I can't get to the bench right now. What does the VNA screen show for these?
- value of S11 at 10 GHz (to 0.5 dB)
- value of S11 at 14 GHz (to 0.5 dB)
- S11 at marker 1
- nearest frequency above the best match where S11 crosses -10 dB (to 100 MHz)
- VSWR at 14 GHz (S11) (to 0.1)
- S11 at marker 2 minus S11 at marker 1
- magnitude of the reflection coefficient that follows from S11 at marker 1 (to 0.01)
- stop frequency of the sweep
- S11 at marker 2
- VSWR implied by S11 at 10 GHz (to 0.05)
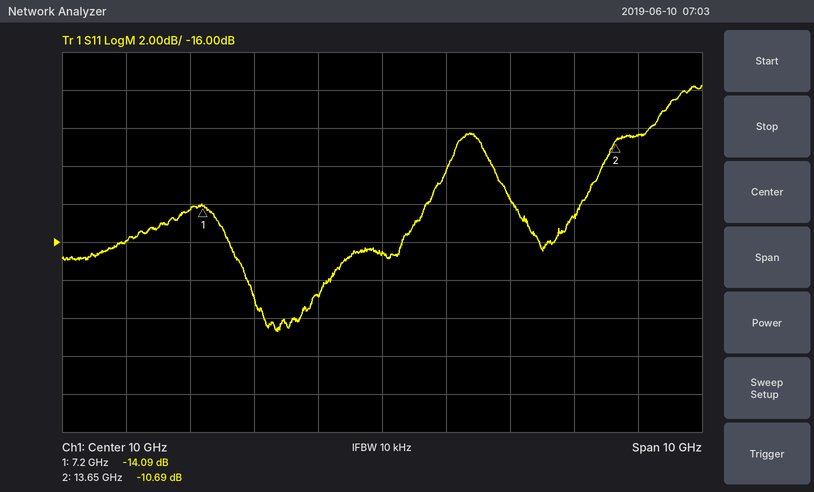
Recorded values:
-16.5 dB
-10.5 dB
-14.09 dB
14.2 GHz
1.9
3.40 dB
0.20
15 GHz
-10.69 dB
1.35
